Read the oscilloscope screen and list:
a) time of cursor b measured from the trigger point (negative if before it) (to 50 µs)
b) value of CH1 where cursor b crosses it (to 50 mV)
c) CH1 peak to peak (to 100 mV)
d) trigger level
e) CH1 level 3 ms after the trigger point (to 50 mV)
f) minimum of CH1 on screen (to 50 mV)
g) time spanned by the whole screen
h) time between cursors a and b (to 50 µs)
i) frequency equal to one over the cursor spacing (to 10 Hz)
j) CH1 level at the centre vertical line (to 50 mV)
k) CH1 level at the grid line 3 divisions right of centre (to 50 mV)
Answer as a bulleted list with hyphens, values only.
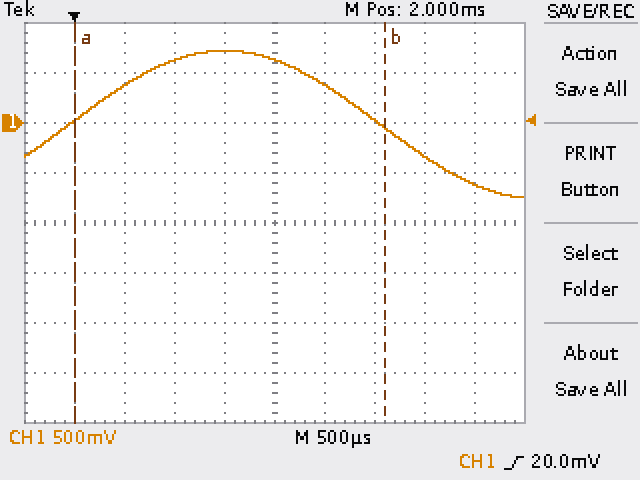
- +3.10 ms
- -50 mV
- 1.50 V
- 20.0 mV
- 50 mV
- -750 mV
- 5 ms
- 3.10 ms
- 320 Hz
- 650 mV
- -350 mV
